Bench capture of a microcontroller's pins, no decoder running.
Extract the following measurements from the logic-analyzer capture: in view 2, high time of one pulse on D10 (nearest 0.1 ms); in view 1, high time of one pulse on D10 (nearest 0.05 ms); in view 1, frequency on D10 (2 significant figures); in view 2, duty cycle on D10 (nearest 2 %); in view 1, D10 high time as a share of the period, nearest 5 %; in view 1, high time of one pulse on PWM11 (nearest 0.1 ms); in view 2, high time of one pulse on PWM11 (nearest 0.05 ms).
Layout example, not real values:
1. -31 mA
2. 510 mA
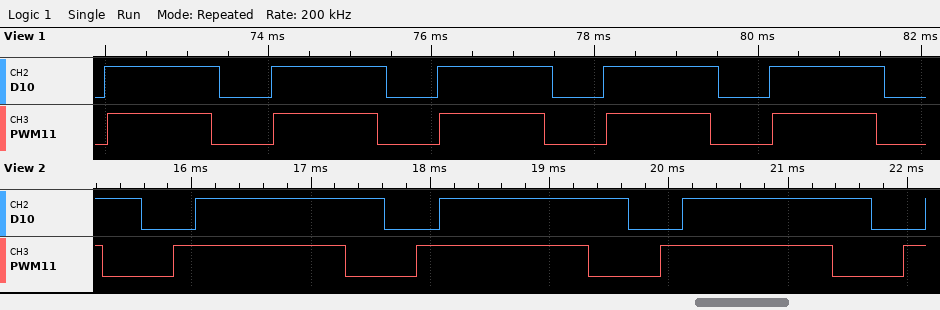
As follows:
1. 1.6 ms
2. 1.40 ms
3. 490 Hz
4. 78 %
5. 70 %
6. 1.3 ms
7. 1.45 ms
